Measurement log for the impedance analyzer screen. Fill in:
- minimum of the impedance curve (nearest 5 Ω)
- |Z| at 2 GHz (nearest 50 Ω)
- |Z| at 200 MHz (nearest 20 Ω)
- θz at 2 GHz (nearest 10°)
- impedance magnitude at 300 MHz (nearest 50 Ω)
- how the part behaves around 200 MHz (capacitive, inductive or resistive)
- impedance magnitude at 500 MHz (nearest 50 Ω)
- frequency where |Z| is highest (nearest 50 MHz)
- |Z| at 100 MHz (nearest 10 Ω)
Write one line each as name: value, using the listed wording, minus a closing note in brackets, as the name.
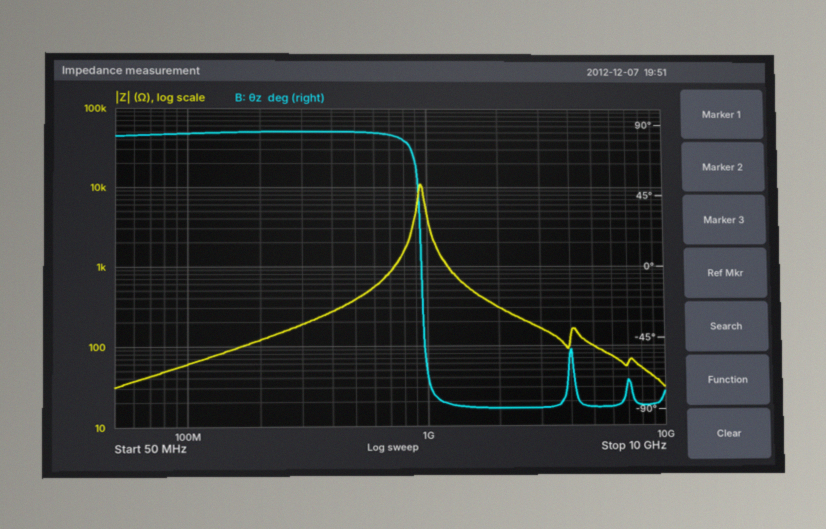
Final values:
minimum of the impedance curve: 30 Ω
|Z| at 2 GHz: 300 Ω
|Z| at 200 MHz: 120 Ω
θz at 2 GHz: -90°
impedance magnitude at 300 MHz: 200 Ω
how the part behaves around 200 MHz: inductive
impedance magnitude at 500 MHz: 400 Ω
frequency where |Z| is highest: 950 MHz
|Z| at 100 MHz: 60 Ω
